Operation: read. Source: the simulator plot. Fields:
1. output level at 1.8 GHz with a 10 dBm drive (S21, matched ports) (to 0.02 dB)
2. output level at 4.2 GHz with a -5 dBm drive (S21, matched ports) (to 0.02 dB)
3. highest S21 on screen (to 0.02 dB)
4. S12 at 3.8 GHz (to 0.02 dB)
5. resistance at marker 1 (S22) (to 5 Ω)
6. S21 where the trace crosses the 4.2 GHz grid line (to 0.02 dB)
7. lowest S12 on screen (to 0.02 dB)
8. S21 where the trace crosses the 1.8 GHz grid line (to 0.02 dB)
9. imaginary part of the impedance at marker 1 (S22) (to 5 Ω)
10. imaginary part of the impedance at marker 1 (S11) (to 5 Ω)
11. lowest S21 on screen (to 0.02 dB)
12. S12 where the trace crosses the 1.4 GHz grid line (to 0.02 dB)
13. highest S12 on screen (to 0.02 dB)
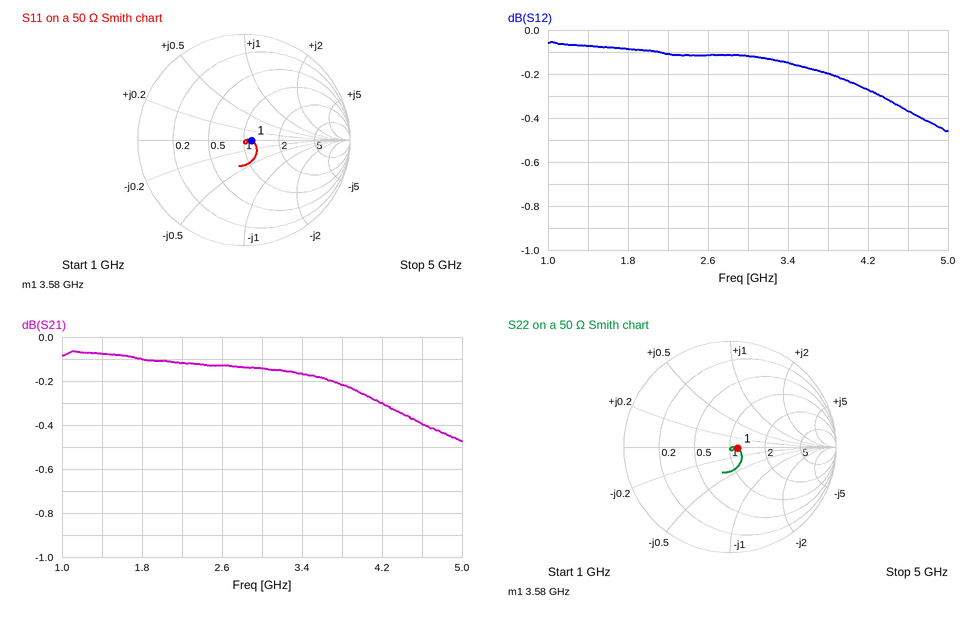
9.90 dBm
-5.30 dBm
-0.06 dB
-0.20 dB
60 Ω
-0.30 dB
-0.46 dB
-0.10 dB
0 Ω
0 Ω
-0.48 dB
-0.08 dB
-0.06 dB
